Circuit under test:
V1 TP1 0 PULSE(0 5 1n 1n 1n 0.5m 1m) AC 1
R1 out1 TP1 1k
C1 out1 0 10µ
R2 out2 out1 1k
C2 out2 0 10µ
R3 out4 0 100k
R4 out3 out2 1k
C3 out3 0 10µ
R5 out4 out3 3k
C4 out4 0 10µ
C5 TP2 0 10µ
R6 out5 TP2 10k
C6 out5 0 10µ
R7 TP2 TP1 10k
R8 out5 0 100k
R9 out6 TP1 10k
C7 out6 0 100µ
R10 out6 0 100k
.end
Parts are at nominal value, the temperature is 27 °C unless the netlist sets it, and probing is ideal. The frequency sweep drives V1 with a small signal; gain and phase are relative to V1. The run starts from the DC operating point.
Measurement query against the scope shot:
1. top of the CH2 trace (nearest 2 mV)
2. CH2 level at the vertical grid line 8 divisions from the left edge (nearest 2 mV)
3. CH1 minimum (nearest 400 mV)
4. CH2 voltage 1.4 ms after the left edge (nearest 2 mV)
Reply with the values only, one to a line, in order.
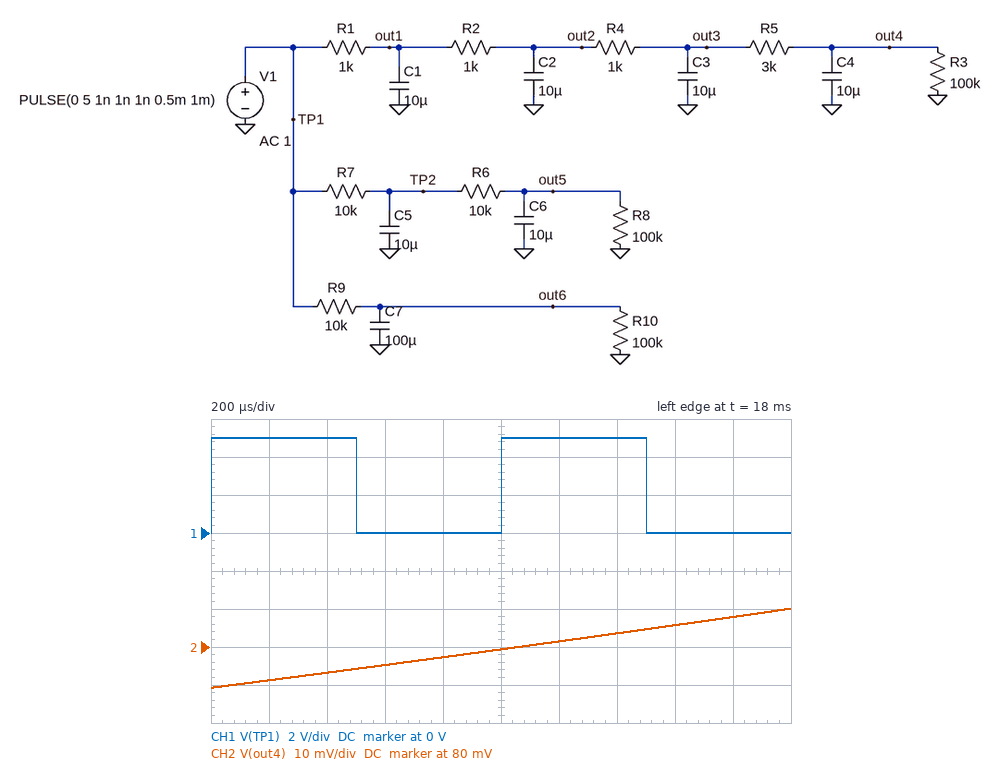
90 mV
86 mV
0 V
84 mV
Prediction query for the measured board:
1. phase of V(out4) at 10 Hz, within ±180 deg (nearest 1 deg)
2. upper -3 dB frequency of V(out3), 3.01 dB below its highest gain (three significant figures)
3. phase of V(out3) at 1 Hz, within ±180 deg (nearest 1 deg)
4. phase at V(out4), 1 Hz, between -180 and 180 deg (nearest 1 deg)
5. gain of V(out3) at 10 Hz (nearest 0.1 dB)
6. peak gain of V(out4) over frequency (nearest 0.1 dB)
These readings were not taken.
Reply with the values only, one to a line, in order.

-159 deg
1.92 Hz
-28 deg
-39 deg
-13.2 dB
-0.5 dB
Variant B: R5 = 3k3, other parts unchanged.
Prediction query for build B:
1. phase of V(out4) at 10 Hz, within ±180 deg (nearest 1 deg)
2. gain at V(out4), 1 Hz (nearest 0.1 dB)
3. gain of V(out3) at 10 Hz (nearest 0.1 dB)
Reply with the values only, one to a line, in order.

-162 deg
-1.8 dB
-13.0 dB
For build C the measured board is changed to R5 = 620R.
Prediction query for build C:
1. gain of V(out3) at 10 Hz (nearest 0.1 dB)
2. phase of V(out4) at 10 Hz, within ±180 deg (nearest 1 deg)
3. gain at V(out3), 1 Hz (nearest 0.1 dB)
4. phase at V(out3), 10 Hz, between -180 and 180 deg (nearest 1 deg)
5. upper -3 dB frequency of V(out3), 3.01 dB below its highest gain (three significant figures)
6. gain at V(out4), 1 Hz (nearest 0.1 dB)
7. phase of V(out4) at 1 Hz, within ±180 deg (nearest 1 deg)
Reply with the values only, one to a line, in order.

-15.2 dB
-129 deg
-1.2 dB
-108 deg
2.00 Hz
-1.3 dB
-32 deg
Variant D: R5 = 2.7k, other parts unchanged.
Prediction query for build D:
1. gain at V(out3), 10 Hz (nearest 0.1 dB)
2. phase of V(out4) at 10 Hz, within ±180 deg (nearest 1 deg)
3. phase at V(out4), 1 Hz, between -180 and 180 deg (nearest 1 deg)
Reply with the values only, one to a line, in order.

-13.4 dB
-157 deg
-38 deg
